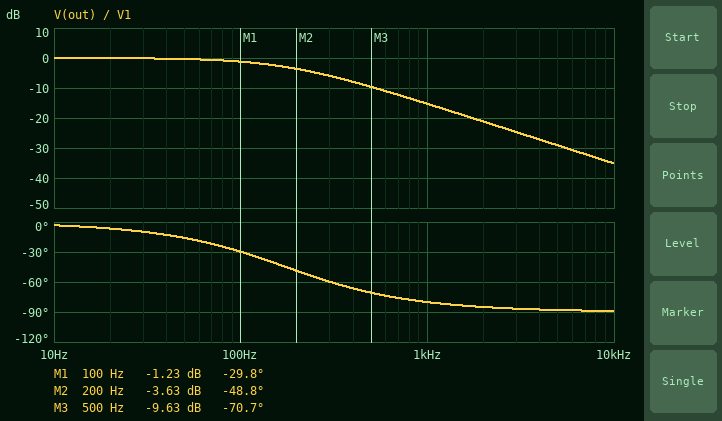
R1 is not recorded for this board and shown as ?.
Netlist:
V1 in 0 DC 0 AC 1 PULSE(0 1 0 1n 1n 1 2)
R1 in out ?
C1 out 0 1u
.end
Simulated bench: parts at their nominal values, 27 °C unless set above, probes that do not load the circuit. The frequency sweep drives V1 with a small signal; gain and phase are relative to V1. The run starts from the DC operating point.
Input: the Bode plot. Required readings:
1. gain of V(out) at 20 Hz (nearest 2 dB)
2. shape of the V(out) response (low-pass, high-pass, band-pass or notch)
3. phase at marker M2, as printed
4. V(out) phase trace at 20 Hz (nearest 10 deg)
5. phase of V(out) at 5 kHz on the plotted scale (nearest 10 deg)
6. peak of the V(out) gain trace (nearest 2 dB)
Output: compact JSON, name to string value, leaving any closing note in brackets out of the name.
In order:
{"gain of V(out) at 20 Hz": "0 dB", "shape of the V(out) response": "low-pass", "phase at marker M2, as printed": "-48.8 deg", "V(out) phase trace at 20 Hz": "-10 deg", "phase of V(out) at 5 kHz on the plotted scale": "-90 deg", "peak of the V(out) gain trace": "0 dB"}
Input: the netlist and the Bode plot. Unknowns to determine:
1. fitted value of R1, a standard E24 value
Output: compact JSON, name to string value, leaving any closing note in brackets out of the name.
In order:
{"fitted value of R1, a standard E24 value": "910 Ω"}
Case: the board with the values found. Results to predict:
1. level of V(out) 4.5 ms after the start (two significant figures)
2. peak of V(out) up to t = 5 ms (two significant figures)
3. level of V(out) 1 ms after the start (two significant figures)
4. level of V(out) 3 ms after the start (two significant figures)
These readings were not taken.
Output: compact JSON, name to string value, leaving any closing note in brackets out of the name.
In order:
{"level of V(out) 4.5 ms after the start": "990 mV", "peak of V(out) up to t = 5 ms": "1.0 V", "level of V(out) 1 ms after the start": "670 mV", "level of V(out) 3 ms after the start": "960 mV"}
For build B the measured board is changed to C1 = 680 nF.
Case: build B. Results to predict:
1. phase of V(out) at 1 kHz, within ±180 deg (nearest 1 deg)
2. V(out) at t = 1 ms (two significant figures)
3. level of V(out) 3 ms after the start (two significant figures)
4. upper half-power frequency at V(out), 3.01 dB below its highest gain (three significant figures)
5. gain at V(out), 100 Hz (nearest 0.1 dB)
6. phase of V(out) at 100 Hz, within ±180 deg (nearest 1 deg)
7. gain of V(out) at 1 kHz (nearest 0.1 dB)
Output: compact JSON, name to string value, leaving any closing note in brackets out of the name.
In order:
{"phase of V(out) at 1 kHz, within ±180 deg": "-76 deg", "V(out) at t = 1 ms": "800 mV", "level of V(out) 3 ms after the start": "990 mV", "upper half-power frequency at V(out), 3.01 dB below its highest gain": "257 Hz", "gain at V(out), 100 Hz": "-0.6 dB", "phase of V(out) at 100 Hz, within ±180 deg": "-21 deg", "gain of V(out) at 1 kHz": "-12.1 dB"}
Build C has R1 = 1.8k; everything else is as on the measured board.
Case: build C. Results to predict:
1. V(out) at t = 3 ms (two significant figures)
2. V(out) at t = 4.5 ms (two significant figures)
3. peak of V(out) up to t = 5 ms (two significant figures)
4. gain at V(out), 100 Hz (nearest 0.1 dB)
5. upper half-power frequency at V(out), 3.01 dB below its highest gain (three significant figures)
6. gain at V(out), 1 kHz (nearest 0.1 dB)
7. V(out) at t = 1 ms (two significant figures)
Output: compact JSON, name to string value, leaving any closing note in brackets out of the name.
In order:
{"V(out) at t = 3 ms": "810 mV", "V(out) at t = 4.5 ms": "920 mV", "peak of V(out) up to t = 5 ms": "940 mV", "gain at V(out), 100 Hz": "-3.6 dB", "upper half-power frequency at V(out), 3.01 dB below its highest gain": "88.4 Hz", "gain at V(out), 1 kHz": "-21.1 dB", "V(out) at t = 1 ms": "430 mV"}
